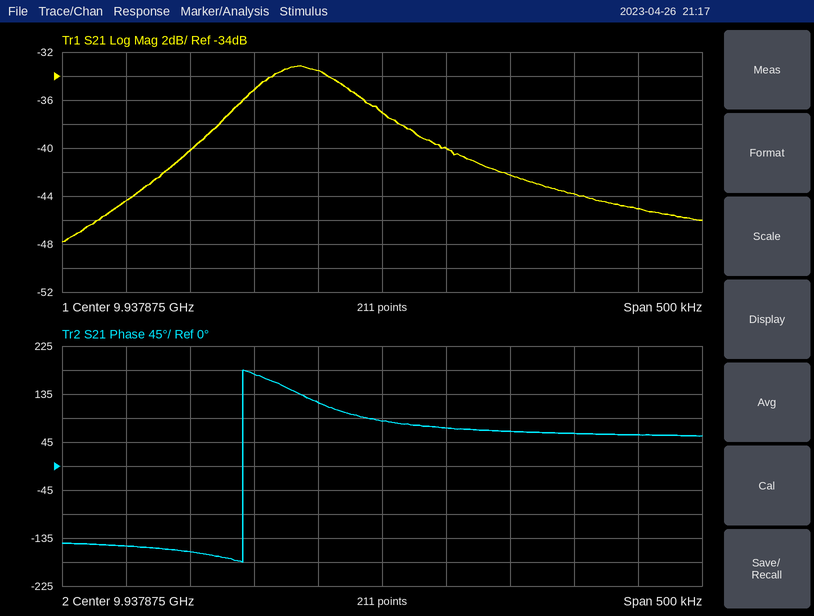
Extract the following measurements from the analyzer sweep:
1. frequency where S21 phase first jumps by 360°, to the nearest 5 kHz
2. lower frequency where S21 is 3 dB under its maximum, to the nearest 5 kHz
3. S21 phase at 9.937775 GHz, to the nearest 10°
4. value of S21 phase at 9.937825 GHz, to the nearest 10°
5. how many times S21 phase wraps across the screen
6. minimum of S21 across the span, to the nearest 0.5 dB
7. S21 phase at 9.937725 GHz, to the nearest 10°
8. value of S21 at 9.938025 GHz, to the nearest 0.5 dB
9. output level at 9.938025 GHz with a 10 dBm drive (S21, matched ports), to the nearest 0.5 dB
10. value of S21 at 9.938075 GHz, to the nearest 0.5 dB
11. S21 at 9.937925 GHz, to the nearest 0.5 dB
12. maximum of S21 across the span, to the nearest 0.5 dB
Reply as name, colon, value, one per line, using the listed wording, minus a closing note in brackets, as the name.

frequency where S21 phase first jumps by 360°, to the nearest 5 kHz: 9.937765 GHz
lower frequency where S21 is 3 dB under its maximum, to the nearest 5 kHz: 9.937765 GHz
S21 phase at 9.937775 GHz, to the nearest 10°: 170°
value of S21 phase at 9.937825 GHz, to the nearest 10°: 120°
how many times S21 phase wraps across the screen: 1
minimum of S21 across the span, to the nearest 0.5 dB: -48.0 dB
S21 phase at 9.937725 GHz, to the nearest 10°: -160°
value of S21 at 9.938025 GHz, to the nearest 0.5 dB: -44.0 dB
output level at 9.938025 GHz with a 10 dBm drive (S21, matched ports), to the nearest 0.5 dB: -34.0 dBm
value of S21 at 9.938075 GHz, to the nearest 0.5 dB: -45.0 dB
S21 at 9.937925 GHz, to the nearest 0.5 dB: -40.0 dB
maximum of S21 across the span, to the nearest 0.5 dB: -33.0 dB
